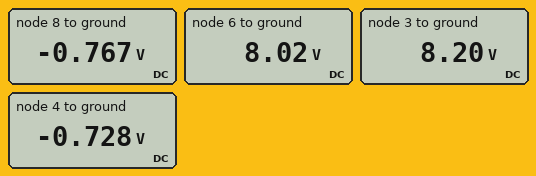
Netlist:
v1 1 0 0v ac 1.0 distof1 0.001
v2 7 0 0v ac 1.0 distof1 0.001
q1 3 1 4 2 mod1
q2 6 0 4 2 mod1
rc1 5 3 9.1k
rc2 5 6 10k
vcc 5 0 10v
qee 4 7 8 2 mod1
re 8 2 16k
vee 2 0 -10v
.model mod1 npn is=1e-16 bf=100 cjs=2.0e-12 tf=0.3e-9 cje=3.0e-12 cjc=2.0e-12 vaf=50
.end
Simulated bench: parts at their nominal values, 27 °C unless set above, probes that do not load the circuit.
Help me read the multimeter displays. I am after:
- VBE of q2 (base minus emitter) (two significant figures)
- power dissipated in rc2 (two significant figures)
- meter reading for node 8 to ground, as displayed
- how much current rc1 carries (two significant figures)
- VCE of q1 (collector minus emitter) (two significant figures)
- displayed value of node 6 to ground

730 mV
390 µW
-0.767 V
200 µA
8.9 V
8.02 V
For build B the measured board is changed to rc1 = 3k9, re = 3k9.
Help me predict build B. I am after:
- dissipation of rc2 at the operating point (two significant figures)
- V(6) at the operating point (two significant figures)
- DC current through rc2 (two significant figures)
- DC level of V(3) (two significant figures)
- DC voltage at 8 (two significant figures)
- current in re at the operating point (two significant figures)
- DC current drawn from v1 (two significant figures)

5.8 mW
2.4 V
760 µA
6.8 V
-800 mV
2.4 mA
7.3 µA
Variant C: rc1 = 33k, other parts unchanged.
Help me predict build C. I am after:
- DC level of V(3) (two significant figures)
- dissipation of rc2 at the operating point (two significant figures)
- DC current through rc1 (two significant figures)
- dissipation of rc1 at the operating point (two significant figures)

3.8 V
410 µW
190 µA
1.2 mW
